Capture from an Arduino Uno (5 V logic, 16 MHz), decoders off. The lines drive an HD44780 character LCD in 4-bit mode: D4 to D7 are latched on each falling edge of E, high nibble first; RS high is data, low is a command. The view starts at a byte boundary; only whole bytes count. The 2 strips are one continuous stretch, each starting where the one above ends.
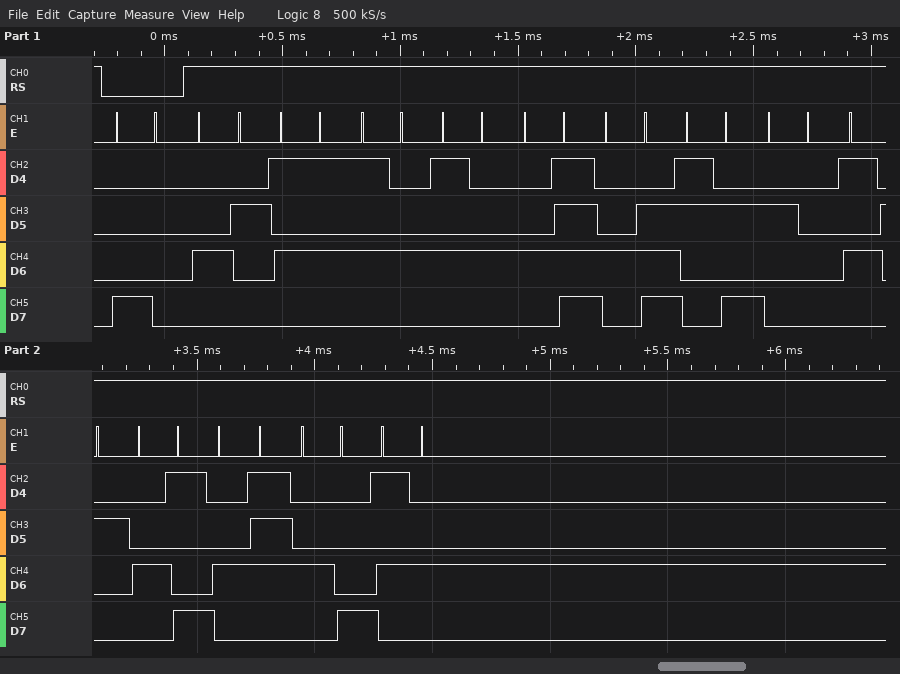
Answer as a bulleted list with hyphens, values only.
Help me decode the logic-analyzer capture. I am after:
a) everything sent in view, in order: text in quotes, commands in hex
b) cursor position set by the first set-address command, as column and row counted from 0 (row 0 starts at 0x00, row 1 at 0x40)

- 0x80 "BUTTON: RIGHT"
- column 0, row 0
